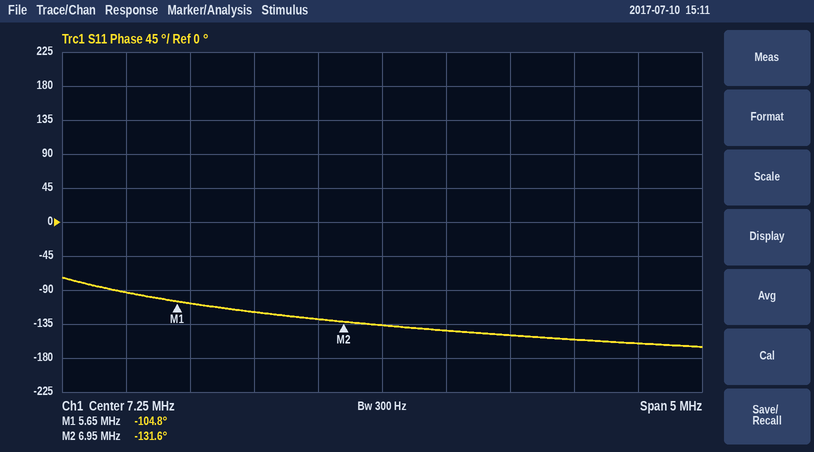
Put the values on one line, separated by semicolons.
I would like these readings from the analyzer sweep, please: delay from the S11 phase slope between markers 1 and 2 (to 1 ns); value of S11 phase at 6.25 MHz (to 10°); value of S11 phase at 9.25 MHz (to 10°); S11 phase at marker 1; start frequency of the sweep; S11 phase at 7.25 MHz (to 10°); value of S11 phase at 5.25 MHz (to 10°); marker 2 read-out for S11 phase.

57 ns; -120°; -160°; -104.8°; 4.75 MHz; -140°; -90°; -131.6°
